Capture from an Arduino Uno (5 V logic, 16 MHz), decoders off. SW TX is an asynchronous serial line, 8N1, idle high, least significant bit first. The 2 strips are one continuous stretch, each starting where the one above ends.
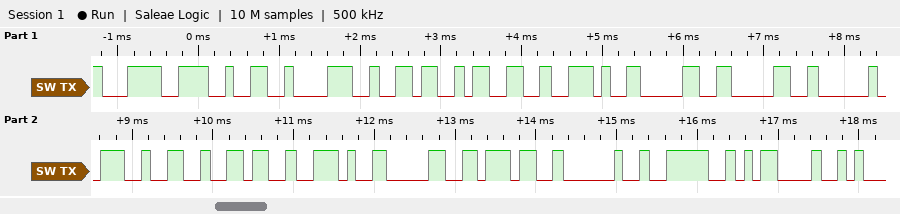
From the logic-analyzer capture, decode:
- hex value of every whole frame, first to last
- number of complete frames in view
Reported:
0x3C 0x32 0x38 0x36 0x33 0x2E 0x30 0x30 0x20 0x32 0x36 0x2E 0x30 0x37 0x20 0x3E 0x0D
17
